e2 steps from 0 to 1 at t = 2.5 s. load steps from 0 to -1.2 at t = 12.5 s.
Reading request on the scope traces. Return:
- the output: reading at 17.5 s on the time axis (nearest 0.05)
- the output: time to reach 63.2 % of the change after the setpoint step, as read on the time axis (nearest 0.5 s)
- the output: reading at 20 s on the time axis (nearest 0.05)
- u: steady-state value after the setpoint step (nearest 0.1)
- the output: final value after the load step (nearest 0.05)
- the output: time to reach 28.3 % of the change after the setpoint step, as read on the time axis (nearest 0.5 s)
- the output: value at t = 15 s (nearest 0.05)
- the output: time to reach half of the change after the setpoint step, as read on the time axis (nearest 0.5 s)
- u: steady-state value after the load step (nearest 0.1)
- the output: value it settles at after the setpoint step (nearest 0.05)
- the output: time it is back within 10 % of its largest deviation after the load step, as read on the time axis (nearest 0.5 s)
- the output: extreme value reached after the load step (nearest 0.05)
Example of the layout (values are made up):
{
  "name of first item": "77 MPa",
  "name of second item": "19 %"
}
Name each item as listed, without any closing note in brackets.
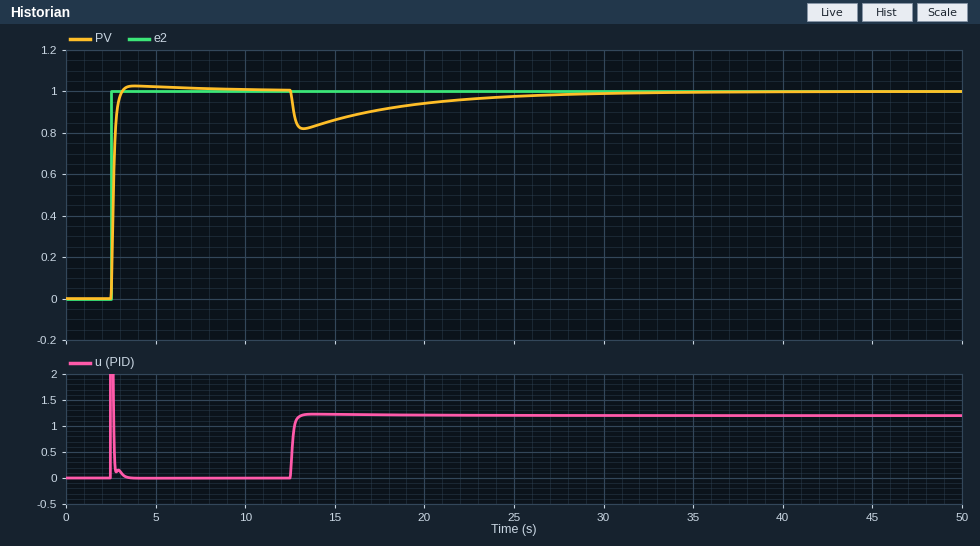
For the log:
{
  "the output: reading at 17.5 s on the time axis": "0.90",
  "the output: time to reach 63.2 % of the change after the setpoint step, as read on the time axis": "2.5 s",
  "the output: reading at 20 s on the time axis": "0.95",
  "u: steady-state value after the setpoint step": "0.0",
  "the output: final value after the load step": "1.00",
  "the output: time to reach 28.3 % of the change after the setpoint step, as read on the time axis": "2.5 s",
  "the output: value at t = 15 s": "0.85",
  "the output: time to reach half of the change after the setpoint step, as read on the time axis": "2.5 s",
  "u: steady-state value after the load step": "1.2",
  "the output: value it settles at after the setpoint step": "1.00",
  "the output: time it is back within 10 % of its largest deviation after the load step, as read on the time axis": "26.5 s",
  "the output: extreme value reached after the load step": "0.80"
}
